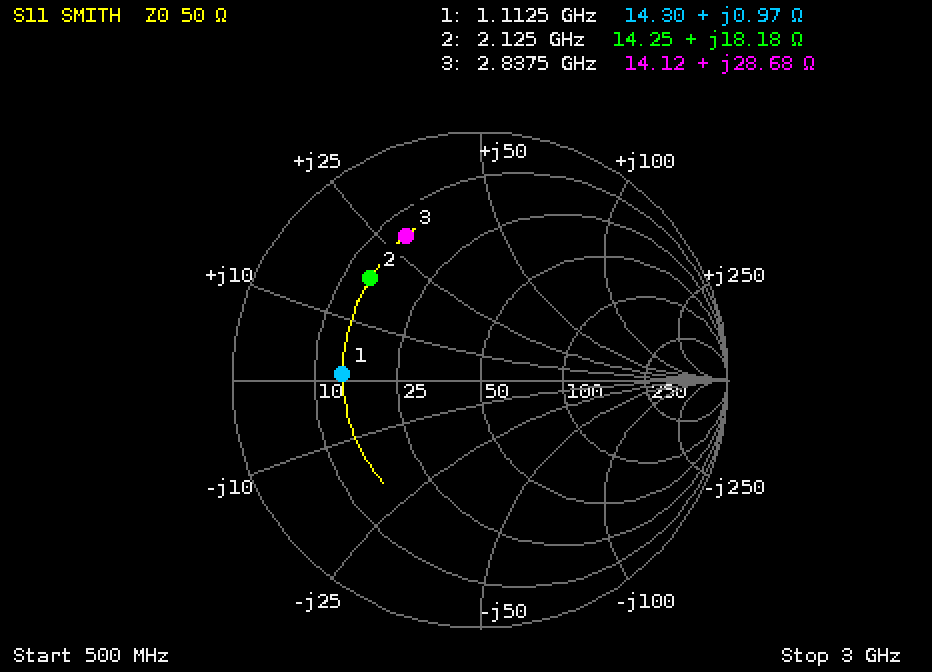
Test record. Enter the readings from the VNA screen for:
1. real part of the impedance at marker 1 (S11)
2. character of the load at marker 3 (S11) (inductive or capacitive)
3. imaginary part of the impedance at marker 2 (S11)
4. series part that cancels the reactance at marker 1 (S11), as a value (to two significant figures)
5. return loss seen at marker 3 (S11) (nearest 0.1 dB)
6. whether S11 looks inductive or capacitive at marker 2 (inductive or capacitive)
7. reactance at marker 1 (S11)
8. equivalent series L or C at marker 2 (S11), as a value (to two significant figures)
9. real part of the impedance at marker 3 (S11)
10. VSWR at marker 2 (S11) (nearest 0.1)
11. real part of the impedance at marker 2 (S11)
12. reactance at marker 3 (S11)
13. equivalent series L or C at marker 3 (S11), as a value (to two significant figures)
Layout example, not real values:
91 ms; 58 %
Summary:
14.30 Ω; inductive; +18.18 Ω; 150 pF; 3.7 dB; inductive; +0.97 Ω; 1.4 nH; 14.12 Ω; 4.0; 14.25 Ω; +28.68 Ω; 1.6 nH
